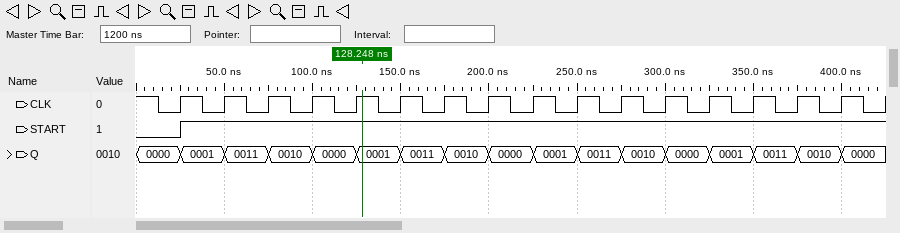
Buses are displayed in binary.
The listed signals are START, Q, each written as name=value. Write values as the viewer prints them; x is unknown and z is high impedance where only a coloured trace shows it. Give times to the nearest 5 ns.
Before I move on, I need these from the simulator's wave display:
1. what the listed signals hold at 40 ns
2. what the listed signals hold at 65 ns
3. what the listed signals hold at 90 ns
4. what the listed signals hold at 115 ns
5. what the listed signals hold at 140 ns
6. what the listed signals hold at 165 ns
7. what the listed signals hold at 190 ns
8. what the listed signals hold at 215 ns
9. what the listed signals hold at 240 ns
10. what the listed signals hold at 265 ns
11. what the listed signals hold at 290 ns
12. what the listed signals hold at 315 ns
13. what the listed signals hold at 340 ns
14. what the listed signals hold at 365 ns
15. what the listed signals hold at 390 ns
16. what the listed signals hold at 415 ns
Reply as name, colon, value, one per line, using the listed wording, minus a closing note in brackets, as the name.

what the listed signals hold at 40 ns: START=1, Q=0001
what the listed signals hold at 65 ns: START=1, Q=0011
what the listed signals hold at 90 ns: START=1, Q=0010
what the listed signals hold at 115 ns: START=1, Q=0000
what the listed signals hold at 140 ns: START=1, Q=0001
what the listed signals hold at 165 ns: START=1, Q=0011
what the listed signals hold at 190 ns: START=1, Q=0010
what the listed signals hold at 215 ns: START=1, Q=0000
what the listed signals hold at 240 ns: START=1, Q=0001
what the listed signals hold at 265 ns: START=1, Q=0011
what the listed signals hold at 290 ns: START=1, Q=0010
what the listed signals hold at 315 ns: START=1, Q=0000
what the listed signals hold at 340 ns: START=1, Q=0001
what the listed signals hold at 365 ns: START=1, Q=0011
what the listed signals hold at 390 ns: START=1, Q=0010
what the listed signals hold at 415 ns: START=1, Q=0000
